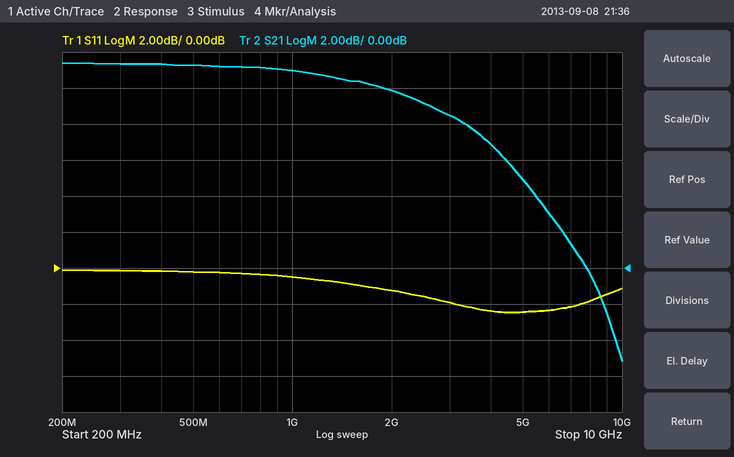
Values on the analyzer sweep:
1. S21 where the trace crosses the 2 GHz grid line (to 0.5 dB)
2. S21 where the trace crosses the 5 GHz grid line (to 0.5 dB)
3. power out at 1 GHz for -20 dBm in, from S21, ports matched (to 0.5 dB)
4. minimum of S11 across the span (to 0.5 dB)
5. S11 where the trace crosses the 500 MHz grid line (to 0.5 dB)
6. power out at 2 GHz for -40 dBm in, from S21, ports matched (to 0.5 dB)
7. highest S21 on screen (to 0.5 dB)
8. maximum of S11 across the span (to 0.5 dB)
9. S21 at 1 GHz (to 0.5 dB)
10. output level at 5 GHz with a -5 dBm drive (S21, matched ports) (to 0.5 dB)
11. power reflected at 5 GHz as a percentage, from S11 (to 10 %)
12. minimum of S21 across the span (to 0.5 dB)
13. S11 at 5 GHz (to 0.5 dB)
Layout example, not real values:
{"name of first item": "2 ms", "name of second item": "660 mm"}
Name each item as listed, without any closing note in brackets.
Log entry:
{"S21 where the trace crosses the 2 GHz grid line": "10.0 dB", "S21 where the trace crosses the 5 GHz grid line": "5.0 dB", "power out at 1 GHz for -20 dBm in, from S21, ports matched": "-9.0 dBm", "minimum of S11 across the span": "-2.5 dB", "S11 where the trace crosses the 500 MHz grid line": "0.0 dB", "power out at 2 GHz for -40 dBm in, from S21, ports matched": "-30.0 dBm", "highest S21 on screen": "11.5 dB", "maximum of S11 across the span": "0.0 dB", "S21 at 1 GHz": "11.0 dB", "output level at 5 GHz with a -5 dBm drive (S21, matched ports)": "0.0 dBm", "power reflected at 5 GHz as a percentage, from S11": "60 %", "minimum of S21 across the span": "-5.0 dB", "S11 at 5 GHz": "-2.5 dB"}
